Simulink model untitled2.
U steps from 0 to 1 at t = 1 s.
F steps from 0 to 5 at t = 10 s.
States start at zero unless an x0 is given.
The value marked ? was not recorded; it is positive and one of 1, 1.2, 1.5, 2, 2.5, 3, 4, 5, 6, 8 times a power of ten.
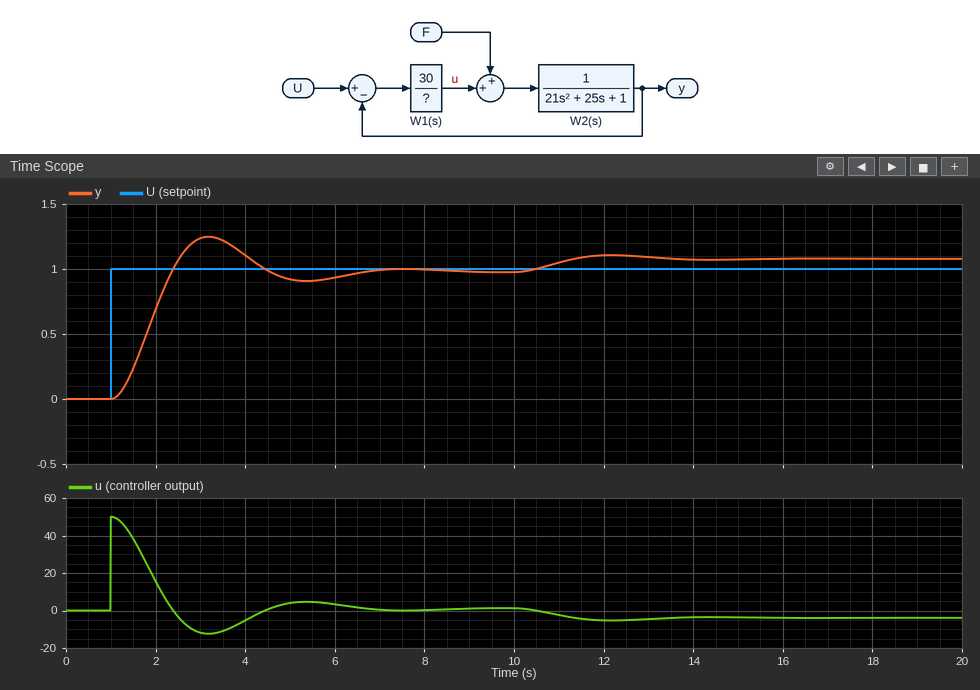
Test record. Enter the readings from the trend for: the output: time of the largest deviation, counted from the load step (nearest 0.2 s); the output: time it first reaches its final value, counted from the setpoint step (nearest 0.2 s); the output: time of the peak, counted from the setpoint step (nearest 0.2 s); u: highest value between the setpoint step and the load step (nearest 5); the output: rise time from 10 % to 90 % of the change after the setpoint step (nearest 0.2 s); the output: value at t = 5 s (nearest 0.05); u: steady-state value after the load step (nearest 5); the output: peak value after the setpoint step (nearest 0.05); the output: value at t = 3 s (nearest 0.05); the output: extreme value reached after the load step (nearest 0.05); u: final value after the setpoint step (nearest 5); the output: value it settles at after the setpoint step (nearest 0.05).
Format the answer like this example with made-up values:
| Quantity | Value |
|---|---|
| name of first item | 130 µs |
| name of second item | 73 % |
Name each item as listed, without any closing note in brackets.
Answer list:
| Quantity | Value |
|---|---|
| the output: time of the largest deviation, counted from the load step | 2.2 s |
| the output: time it first reaches its final value, counted from the setpoint step | 1.4 s |
| the output: time of the peak, counted from the setpoint step | 2.2 s |
| u: highest value between the setpoint step and the load step | 50 |
| the output: rise time from 10 % to 90 % of the change after the setpoint step | 1.0 s |
| the output: value at t = 5 s | 0.90 |
| u: steady-state value after the load step | -5 |
| the output: peak value after the setpoint step | 1.25 |
| the output: value at t = 3 s | 1.25 |
| the output: extreme value reached after the load step | 1.10 |
| u: final value after the setpoint step | 0 |
| the output: value it settles at after the setpoint step | 1.00 |
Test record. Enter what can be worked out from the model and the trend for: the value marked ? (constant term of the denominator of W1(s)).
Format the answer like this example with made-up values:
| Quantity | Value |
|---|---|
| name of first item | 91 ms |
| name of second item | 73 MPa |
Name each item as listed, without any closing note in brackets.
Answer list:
| Quantity | Value |
|---|---|
| the value marked ? (constant term of the denominator of W1(s)) | 0.6 |
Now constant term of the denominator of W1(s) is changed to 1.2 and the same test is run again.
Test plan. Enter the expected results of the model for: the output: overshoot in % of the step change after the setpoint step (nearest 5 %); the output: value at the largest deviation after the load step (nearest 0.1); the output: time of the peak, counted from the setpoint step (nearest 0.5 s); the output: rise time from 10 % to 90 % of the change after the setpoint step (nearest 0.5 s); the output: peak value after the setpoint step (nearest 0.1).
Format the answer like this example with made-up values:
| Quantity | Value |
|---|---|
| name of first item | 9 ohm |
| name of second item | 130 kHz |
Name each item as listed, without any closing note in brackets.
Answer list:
| Quantity | Value |
|---|---|
| the output: overshoot in % of the step change after the setpoint step | 15 % |
| the output: value at the largest deviation after the load step | 1.2 |
| the output: time of the peak, counted from the setpoint step | 3.5 s |
| the output: rise time from 10 % to 90 % of the change after the setpoint step | 1.5 s |
| the output: peak value after the setpoint step | 1.1 |
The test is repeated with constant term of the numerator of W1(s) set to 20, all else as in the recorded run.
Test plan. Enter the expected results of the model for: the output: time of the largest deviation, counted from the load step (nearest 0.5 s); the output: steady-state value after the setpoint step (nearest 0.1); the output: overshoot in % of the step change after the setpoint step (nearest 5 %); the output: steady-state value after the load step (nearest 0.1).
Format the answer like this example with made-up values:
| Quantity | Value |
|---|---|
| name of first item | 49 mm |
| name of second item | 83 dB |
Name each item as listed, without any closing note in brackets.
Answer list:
| Quantity | Value |
|---|---|
| the output: time of the largest deviation, counted from the load step | 3.0 s |
| the output: steady-state value after the setpoint step | 1.0 |
| the output: overshoot in % of the step change after the setpoint step | 20 % |
| the output: steady-state value after the load step | 1.1 |
